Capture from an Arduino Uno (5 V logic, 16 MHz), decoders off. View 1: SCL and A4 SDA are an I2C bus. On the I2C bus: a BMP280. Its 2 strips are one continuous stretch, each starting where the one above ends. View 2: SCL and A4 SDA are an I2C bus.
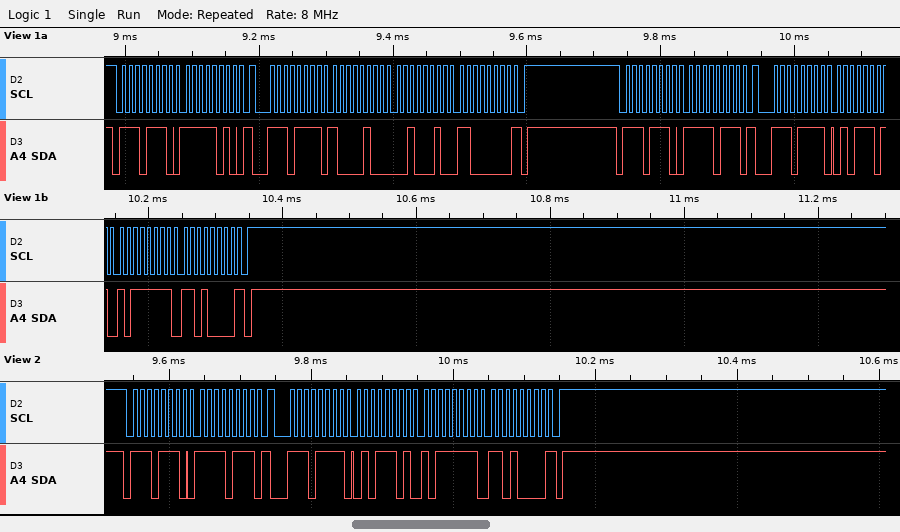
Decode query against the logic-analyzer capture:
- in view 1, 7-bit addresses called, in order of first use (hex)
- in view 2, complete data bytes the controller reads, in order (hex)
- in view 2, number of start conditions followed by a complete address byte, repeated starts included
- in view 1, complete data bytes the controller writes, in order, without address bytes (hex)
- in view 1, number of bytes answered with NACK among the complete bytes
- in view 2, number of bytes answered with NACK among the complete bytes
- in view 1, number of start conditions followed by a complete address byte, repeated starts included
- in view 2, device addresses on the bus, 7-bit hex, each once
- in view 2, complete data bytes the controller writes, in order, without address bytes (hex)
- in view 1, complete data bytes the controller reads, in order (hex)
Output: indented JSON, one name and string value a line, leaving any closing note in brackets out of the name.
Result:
{
  "in view 1, 7-bit addresses called, in order of first use": "0x77",
  "in view 2, complete data bytes the controller reads, in order": "5D BF D0",
  "in view 2, number of start conditions followed by a complete address byte, repeated starts included": "2",
  "in view 1, complete data bytes the controller writes, in order, without address bytes": "FA F7",
  "in view 1, number of bytes answered with NACK among the complete bytes": "2",
  "in view 2, number of bytes answered with NACK among the complete bytes": "1",
  "in view 1, number of start conditions followed by a complete address byte, repeated starts included": "4",
  "in view 2, device addresses on the bus, 7-bit hex, each once": "0x77",
  "in view 2, complete data bytes the controller writes, in order, without address bytes": "F7",
  "in view 1, complete data bytes the controller reads, in order": "84 22 C0 5D BF D0"
}
